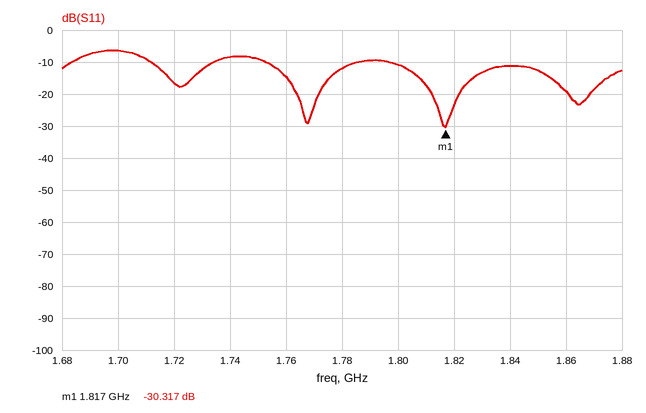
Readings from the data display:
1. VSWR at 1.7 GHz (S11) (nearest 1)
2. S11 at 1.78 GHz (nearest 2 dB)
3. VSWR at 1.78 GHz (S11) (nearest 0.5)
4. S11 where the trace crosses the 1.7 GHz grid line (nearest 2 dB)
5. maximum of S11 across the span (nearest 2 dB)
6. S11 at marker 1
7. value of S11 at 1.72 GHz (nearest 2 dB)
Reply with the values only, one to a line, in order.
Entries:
3
-12 dB
1.5
-6 dB
-6 dB
-30.317 dB
-16 dB
